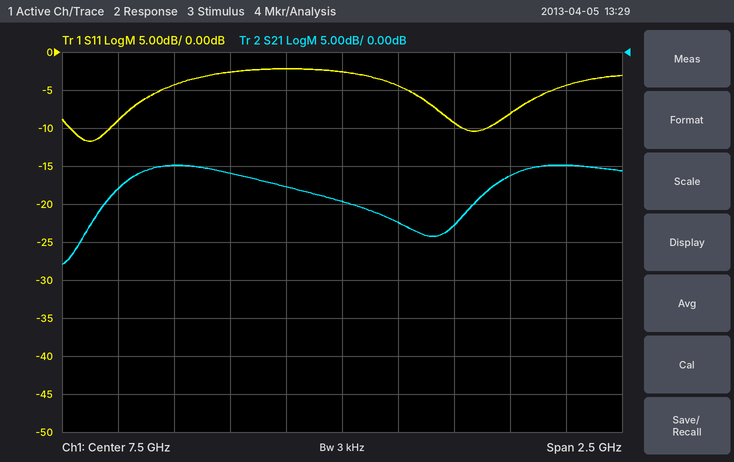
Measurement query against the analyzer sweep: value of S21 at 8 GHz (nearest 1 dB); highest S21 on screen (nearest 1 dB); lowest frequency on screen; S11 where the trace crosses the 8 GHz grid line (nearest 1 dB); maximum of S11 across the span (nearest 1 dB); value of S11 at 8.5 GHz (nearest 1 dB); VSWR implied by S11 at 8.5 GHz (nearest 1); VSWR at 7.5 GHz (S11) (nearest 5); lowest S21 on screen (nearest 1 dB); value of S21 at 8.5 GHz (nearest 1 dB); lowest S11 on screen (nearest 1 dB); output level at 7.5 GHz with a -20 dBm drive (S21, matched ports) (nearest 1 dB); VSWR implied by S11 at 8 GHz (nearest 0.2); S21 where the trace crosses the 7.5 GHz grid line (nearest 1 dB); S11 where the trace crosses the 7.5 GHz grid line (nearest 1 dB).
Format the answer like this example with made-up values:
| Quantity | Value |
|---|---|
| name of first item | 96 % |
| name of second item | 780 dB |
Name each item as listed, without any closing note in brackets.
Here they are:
| Quantity | Value |
|---|---|
| value of S21 at 8 GHz | -23 dB |
| highest S21 on screen | -15 dB |
| lowest frequency on screen | 6.25 GHz |
| S11 where the trace crosses the 8 GHz grid line | -9 dB |
| maximum of S11 across the span | -2 dB |
| value of S11 at 8.5 GHz | -4 dB |
| VSWR implied by S11 at 8.5 GHz | 4 |
| VSWR at 7.5 GHz (S11) | 5 |
| lowest S21 on screen | -28 dB |
| value of S21 at 8.5 GHz | -15 dB |
| lowest S11 on screen | -12 dB |
| output level at 7.5 GHz with a -20 dBm drive (S21, matched ports) | -40 dBm |
| VSWR implied by S11 at 8 GHz | 2.0 |
| S21 where the trace crosses the 7.5 GHz grid line | -20 dB |
| S11 where the trace crosses the 7.5 GHz grid line | -3 dB |
